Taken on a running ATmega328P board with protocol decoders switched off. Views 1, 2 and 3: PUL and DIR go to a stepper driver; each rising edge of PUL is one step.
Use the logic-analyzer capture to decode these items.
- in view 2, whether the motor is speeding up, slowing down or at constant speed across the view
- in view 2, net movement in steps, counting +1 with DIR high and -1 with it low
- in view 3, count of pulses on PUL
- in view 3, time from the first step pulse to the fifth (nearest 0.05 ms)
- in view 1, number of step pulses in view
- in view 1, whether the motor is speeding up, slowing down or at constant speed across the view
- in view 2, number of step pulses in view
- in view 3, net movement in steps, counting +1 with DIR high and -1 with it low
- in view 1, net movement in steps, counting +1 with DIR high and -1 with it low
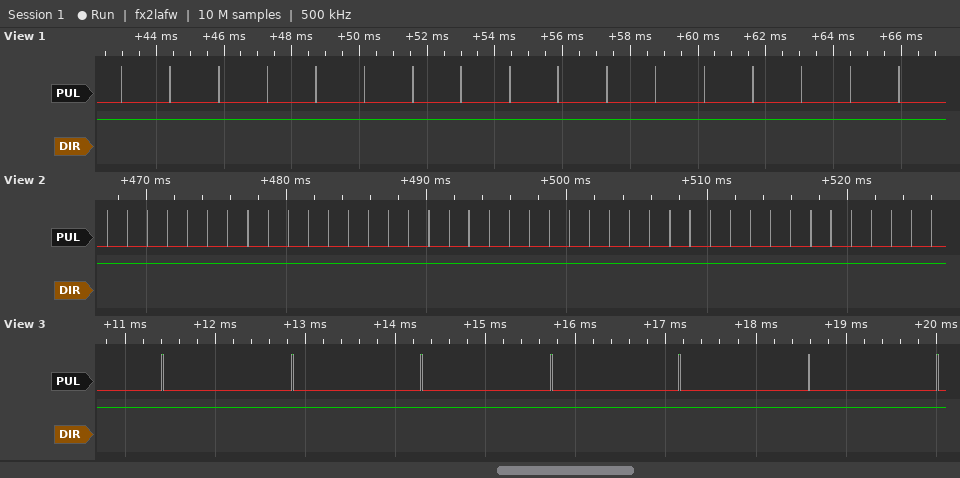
constant speed
+42
7
5.75 ms
17
constant speed
42
+7
+17
